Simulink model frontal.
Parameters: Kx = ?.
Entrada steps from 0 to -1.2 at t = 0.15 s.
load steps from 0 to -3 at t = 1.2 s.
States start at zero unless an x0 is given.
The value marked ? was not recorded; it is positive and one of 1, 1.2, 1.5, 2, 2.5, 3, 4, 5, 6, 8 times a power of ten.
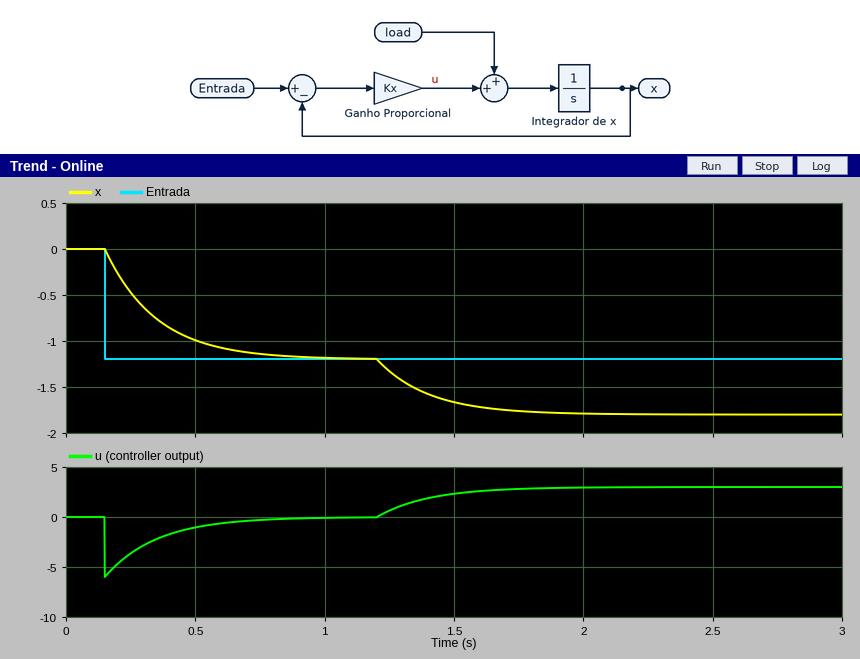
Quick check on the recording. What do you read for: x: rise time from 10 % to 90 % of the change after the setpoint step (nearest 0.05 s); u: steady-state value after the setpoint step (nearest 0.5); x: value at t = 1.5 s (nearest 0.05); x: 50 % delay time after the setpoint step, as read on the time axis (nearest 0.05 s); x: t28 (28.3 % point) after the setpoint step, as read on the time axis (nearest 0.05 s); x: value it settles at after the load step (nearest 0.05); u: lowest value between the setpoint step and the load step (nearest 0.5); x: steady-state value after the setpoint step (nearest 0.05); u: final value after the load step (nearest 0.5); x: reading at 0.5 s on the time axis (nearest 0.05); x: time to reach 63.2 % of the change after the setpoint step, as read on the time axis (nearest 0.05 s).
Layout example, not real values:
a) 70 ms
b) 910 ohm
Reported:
a) 0.45 s
b) 0.0
c) -1.65
d) 0.30 s
e) 0.20 s
f) -1.80
g) -6.0
h) -1.20
i) 3.0
j) -1.00
k) 0.35 s
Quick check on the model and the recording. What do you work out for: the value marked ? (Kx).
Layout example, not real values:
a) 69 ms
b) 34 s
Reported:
a) 5
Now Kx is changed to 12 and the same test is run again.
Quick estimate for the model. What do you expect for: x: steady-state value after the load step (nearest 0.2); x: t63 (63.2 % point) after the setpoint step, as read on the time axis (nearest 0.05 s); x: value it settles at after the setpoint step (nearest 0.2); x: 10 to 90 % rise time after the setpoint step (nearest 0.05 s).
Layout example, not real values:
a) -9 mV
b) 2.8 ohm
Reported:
a) -1.4
b) 0.25 s
c) -1.2
d) 0.20 s
